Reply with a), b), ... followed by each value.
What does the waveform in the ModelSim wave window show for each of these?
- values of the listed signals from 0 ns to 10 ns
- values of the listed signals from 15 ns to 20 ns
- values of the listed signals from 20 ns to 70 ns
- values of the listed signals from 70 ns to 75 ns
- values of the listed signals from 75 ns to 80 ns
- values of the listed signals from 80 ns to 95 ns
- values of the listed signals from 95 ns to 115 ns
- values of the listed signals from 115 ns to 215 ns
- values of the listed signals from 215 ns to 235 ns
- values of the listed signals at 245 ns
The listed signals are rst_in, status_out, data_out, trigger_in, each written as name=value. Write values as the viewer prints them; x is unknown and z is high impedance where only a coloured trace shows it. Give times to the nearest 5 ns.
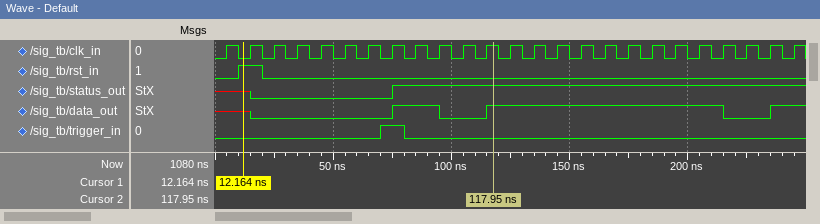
a) rst_in=0, status_out=x, data_out=x, trigger_in=0
b) rst_in=1, status_out=0, data_out=0, trigger_in=0
c) rst_in=0, status_out=0, data_out=0, trigger_in=0
d) rst_in=0, status_out=0, data_out=0, trigger_in=1
e) rst_in=0, status_out=1, data_out=1, trigger_in=1
f) rst_in=0, status_out=1, data_out=1, trigger_in=0
g) rst_in=0, status_out=1, data_out=0, trigger_in=0
h) rst_in=0, status_out=1, data_out=1, trigger_in=0
i) rst_in=0, status_out=1, data_out=0, trigger_in=0
j) rst_in=0, status_out=1, data_out=1, trigger_in=0
